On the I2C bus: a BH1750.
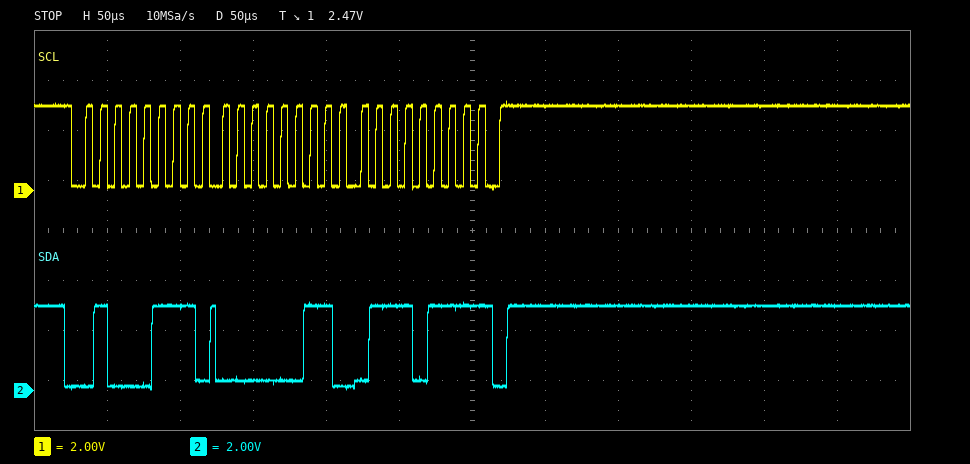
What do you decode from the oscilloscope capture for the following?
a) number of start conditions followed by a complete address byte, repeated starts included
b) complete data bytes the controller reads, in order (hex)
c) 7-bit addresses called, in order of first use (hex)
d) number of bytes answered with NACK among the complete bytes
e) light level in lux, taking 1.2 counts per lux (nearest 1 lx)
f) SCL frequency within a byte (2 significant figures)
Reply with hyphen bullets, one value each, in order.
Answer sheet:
- 1
- 03 77
- 0x23
- 1
- 739 lx
- 100 kHz
